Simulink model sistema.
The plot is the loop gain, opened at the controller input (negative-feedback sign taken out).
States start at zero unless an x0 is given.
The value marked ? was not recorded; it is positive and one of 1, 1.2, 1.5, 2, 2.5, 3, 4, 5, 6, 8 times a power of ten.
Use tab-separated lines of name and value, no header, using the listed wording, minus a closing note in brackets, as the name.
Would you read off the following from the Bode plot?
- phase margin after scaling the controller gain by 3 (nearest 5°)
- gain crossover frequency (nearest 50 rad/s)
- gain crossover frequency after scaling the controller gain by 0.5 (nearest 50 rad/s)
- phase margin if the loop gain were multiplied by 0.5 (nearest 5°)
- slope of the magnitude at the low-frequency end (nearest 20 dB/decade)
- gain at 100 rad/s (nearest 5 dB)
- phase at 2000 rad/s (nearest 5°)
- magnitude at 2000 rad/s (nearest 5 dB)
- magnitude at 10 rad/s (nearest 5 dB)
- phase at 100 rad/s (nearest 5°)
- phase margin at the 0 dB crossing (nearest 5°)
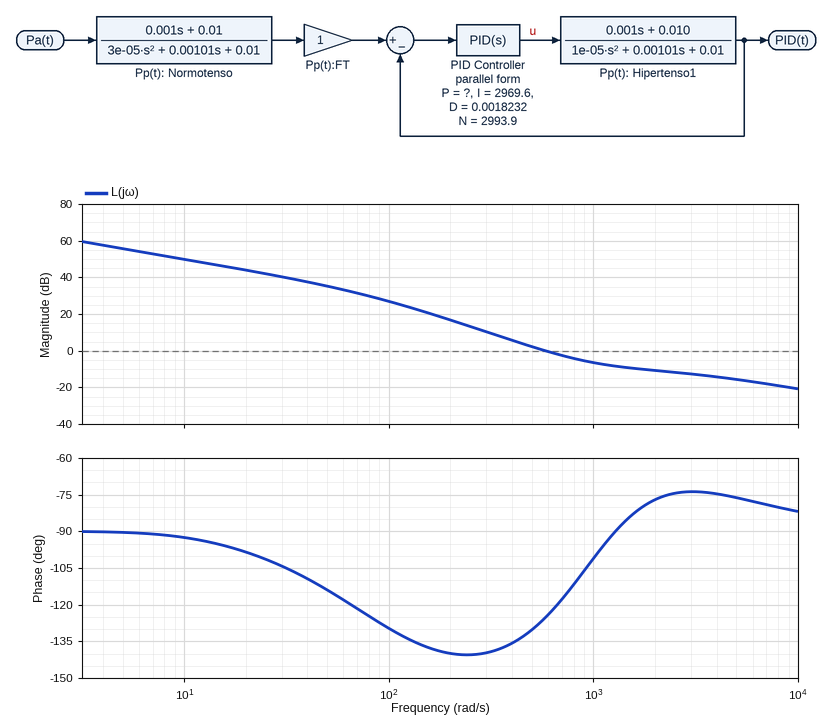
phase margin after scaling the controller gain by 3	95°
gain crossover frequency	600 rad/s
gain crossover frequency after scaling the controller gain by 0.5	400 rad/s
phase margin if the loop gain were multiplied by 0.5	45°
slope of the magnitude at the low-frequency end	-20 dB/decade
gain at 100 rad/s	25 dB
phase at 2000 rad/s	-75°
magnitude at 2000 rad/s	-10 dB
magnitude at 10 rad/s	50 dB
phase at 100 rad/s	-130°
phase margin at the 0 dB crossing	55°
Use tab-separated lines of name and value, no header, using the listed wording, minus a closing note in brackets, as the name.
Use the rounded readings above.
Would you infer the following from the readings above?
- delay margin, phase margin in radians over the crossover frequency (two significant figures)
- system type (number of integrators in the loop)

delay margin, phase margin in radians over the crossover frequency	0.0016 s
system type	1
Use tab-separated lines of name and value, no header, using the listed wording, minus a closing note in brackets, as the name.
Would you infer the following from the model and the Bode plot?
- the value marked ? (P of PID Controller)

the value marked ?	4
